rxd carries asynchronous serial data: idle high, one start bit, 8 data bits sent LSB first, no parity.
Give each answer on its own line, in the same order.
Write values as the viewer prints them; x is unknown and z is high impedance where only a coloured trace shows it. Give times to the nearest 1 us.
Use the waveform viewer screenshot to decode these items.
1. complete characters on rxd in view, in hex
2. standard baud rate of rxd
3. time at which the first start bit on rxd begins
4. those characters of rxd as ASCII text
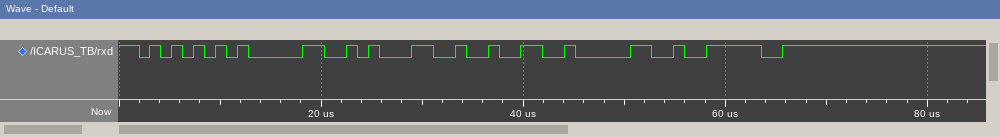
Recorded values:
55, 30, 31, 32, 30, 3E
921600 baud
2 us
"U0120>"
